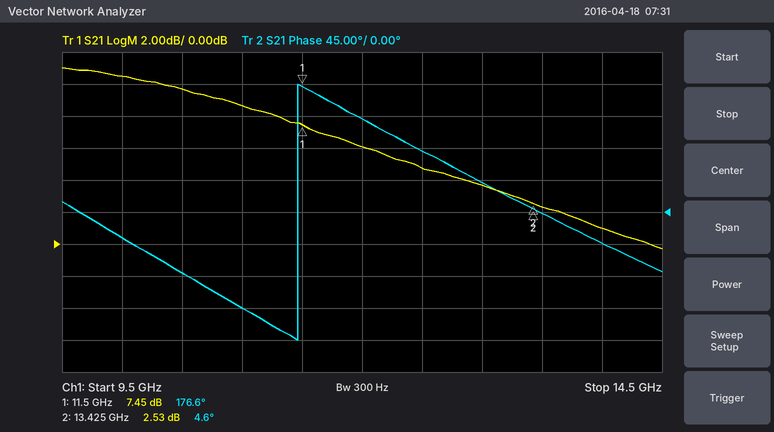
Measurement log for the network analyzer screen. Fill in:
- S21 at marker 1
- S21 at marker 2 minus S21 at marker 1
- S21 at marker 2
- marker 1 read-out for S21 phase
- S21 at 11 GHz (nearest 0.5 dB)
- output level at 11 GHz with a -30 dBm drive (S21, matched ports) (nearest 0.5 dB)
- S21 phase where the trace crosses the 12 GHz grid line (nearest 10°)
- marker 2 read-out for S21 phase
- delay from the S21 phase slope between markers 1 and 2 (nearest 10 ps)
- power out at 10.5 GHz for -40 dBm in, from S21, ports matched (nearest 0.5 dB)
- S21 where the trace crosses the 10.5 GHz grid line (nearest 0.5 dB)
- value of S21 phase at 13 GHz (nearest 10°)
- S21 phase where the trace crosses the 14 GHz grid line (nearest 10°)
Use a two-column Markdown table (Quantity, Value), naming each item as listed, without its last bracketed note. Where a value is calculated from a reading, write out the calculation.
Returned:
| Quantity | Value |
|---|---|
| S21 at marker 1 | 7.45 dB |
| S21 at marker 2 minus S21 at marker 1 | 2.53 − (7.45) = -4.92 dB |
| S21 at marker 2 | 2.53 dB |
| marker 1 read-out for S21 phase | 176.6° |
| S21 at 11 GHz | 8.5 dB |
| output level at 11 GHz with a -30 dBm drive (S21, matched ports) | -30 dBm + (8.5 dB) = -21.5 dBm |
| S21 phase where the trace crosses the 12 GHz grid line | 130° |
| marker 2 read-out for S21 phase | 4.6° |
| delay from the S21 phase slope between markers 1 and 2 | −(4.6° − (176.6°))/(360° × 1.925 GHz) ≈ 248 ps, so 250 ps to the nearest 10 ps |
| power out at 10.5 GHz for -40 dBm in, from S21, ports matched | -40 dBm + (9.5 dB) = -30.5 dBm |
| S21 where the trace crosses the 10.5 GHz grid line | 9.5 dB |
| value of S21 phase at 13 GHz | 40° |
| S21 phase where the trace crosses the 14 GHz grid line | -40° |
